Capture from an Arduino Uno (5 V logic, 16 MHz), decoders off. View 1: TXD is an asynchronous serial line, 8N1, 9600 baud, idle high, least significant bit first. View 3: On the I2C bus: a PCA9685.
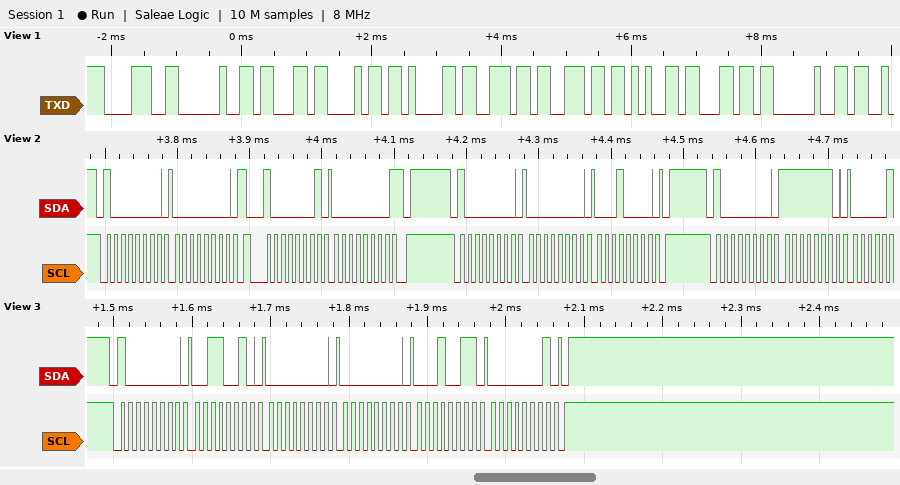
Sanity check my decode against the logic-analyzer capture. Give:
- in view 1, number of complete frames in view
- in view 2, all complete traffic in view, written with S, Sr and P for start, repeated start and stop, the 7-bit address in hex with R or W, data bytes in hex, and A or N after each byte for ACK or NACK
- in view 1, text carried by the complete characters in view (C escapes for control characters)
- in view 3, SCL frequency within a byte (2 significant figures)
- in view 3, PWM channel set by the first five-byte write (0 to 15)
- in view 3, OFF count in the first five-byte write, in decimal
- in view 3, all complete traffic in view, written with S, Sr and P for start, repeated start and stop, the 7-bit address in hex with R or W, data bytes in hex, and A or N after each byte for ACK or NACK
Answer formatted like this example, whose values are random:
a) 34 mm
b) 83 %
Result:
a) 10
b) S 40W A 00 A Sr 40R A 00 N P S 40W A 00 A 10 A P S 40W A FE A
c) "8 channel "
d) 100 kHz
e) 11
f) 275
g) S 40W A 32 A 00 A 00 A 13 A 01 A P
